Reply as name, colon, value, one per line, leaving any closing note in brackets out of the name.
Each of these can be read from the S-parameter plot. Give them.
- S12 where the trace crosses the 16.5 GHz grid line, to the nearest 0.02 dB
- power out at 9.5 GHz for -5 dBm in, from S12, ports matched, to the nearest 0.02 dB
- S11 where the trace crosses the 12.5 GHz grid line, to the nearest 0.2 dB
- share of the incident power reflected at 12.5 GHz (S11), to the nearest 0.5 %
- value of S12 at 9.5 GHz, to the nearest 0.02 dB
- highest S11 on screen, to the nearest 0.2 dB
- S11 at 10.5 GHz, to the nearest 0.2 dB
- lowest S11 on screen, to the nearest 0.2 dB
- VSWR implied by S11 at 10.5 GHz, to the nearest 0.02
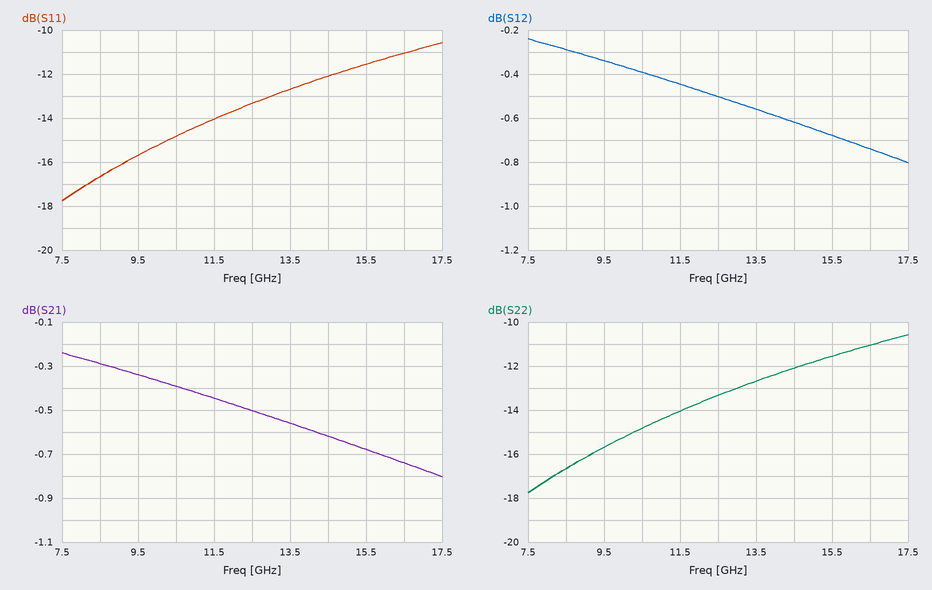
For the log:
S12 where the trace crosses the 16.5 GHz grid line, to the nearest 0.02 dB: -0.74 dB
power out at 9.5 GHz for -5 dBm in, from S12, ports matched, to the nearest 0.02 dB: -5.34 dBm
S11 where the trace crosses the 12.5 GHz grid line, to the nearest 0.2 dB: -13.4 dB
share of the incident power reflected at 12.5 GHz (S11), to the nearest 0.5 %: 4.5 %
value of S12 at 9.5 GHz, to the nearest 0.02 dB: -0.34 dB
highest S11 on screen, to the nearest 0.2 dB: -10.6 dB
S11 at 10.5 GHz, to the nearest 0.2 dB: -14.8 dB
lowest S11 on screen, to the nearest 0.2 dB: -17.8 dB
VSWR implied by S11 at 10.5 GHz, to the nearest 0.02: 1.44
